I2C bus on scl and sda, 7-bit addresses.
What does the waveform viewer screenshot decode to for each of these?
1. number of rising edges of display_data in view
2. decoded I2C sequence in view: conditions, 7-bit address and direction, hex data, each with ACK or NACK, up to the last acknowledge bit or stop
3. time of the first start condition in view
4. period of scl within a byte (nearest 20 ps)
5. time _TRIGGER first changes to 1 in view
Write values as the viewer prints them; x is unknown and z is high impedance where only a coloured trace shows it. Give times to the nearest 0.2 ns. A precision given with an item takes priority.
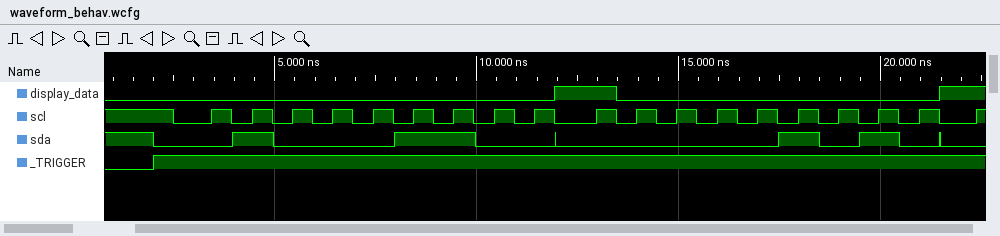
2
start, address 23 write ACK, 05 ACK
2 ns
1000 ps
2 ns
